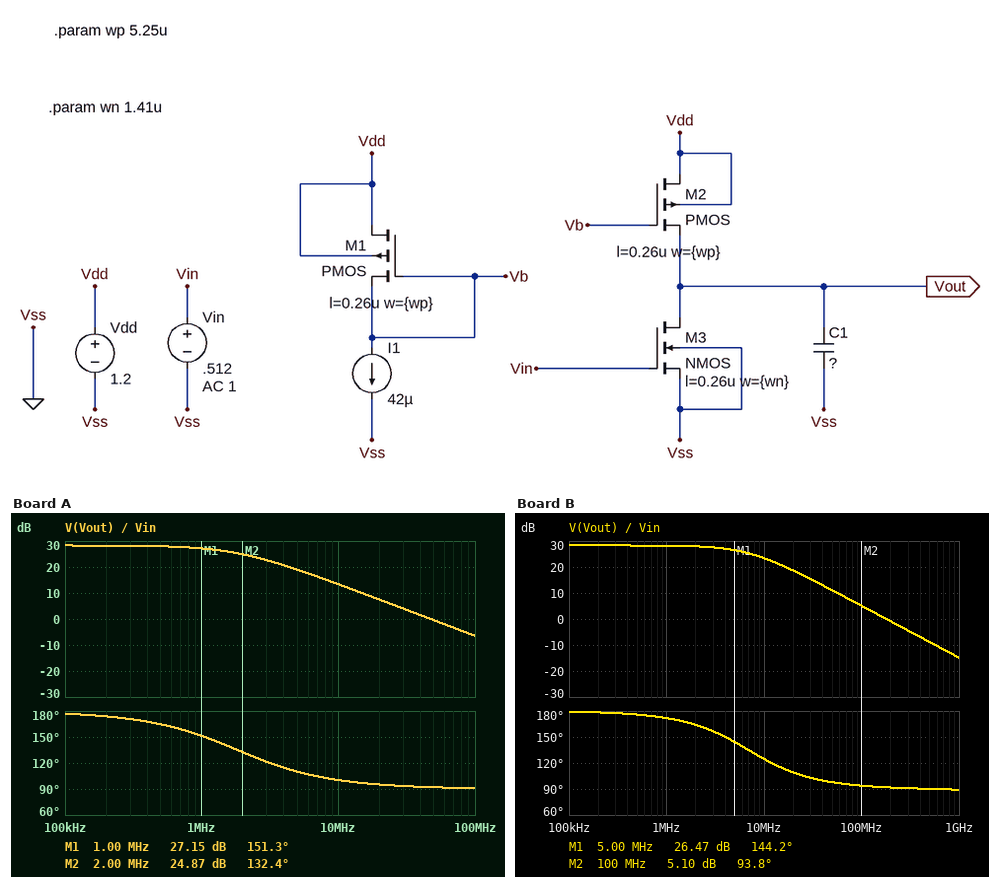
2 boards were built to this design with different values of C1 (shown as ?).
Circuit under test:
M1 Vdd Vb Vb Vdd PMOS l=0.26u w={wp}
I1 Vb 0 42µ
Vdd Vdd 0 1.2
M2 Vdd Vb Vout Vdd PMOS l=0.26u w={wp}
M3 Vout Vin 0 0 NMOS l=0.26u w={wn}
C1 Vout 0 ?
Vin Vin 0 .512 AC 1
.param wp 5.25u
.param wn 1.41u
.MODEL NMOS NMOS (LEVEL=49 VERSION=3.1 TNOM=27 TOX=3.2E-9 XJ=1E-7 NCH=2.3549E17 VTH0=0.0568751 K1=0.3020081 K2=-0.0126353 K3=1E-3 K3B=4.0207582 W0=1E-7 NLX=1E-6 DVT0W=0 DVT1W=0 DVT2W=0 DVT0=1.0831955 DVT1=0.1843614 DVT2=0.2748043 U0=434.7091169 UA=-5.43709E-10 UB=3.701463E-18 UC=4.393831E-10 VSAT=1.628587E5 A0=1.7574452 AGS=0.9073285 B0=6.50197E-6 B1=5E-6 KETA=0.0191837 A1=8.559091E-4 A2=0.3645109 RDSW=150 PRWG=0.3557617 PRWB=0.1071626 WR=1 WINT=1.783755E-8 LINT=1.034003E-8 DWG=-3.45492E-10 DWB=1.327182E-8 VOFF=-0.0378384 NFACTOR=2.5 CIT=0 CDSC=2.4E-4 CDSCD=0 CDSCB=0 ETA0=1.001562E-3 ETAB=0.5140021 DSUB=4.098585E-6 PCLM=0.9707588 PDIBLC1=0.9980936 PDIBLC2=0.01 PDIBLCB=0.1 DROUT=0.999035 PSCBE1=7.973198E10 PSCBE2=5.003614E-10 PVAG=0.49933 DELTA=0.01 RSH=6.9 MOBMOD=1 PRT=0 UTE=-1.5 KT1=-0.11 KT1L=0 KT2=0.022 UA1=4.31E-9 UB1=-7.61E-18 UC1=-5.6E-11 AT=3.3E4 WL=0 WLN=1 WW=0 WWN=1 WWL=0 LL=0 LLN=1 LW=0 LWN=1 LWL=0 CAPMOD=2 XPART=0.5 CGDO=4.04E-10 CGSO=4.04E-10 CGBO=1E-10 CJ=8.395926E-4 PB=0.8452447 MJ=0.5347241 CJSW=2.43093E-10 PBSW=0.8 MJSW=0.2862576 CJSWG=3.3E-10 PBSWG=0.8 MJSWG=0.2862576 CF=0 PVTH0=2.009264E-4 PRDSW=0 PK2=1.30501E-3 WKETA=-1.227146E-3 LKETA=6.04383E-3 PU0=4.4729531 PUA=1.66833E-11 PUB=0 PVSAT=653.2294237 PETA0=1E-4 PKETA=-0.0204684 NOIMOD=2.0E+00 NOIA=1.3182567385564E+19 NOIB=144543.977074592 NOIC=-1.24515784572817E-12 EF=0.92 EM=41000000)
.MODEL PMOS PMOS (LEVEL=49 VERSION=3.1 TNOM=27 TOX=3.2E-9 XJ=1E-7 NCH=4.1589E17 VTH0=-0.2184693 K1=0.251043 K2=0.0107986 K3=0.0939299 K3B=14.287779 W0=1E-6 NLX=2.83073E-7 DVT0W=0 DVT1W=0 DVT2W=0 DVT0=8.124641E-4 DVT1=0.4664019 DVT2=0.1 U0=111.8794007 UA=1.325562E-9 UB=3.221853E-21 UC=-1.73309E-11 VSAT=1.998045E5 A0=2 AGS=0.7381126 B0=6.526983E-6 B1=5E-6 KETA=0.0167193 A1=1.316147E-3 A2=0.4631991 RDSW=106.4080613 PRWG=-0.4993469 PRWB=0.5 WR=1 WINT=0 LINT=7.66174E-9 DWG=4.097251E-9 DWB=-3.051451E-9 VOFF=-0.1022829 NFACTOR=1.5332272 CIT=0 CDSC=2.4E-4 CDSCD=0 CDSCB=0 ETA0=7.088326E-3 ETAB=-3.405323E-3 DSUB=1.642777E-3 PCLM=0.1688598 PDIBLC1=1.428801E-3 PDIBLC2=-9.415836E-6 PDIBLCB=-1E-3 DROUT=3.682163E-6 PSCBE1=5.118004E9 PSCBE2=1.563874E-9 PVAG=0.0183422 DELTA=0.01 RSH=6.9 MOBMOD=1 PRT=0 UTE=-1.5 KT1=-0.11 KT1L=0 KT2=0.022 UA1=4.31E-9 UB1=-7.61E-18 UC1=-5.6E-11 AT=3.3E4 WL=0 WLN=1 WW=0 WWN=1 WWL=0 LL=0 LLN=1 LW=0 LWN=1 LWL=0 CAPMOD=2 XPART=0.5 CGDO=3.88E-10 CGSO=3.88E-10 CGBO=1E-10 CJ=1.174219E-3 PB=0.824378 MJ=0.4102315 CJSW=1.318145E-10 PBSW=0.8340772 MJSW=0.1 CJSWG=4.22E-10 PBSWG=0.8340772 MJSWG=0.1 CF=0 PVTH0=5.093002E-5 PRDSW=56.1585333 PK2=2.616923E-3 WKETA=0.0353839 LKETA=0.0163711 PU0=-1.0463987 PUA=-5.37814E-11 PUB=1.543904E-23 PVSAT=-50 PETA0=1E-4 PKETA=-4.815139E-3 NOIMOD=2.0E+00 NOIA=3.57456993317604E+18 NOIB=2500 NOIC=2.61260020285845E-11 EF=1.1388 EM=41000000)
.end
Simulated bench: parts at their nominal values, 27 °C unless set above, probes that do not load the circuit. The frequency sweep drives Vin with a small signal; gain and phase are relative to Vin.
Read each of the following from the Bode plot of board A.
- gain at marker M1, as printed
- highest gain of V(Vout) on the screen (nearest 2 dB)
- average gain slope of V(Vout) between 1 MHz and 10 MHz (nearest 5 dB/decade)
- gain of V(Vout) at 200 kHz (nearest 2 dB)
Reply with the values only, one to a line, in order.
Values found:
27.15 dB
28 dB
-15 dB/decade
28 dB
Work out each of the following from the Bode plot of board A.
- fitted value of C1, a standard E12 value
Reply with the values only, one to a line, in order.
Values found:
1.5 pF
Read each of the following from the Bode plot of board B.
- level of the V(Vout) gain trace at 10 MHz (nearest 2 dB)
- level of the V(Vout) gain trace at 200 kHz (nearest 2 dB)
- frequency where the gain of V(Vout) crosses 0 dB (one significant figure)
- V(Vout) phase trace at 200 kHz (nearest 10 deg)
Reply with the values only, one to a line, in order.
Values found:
24 dB
28 dB
200 MHz
180 deg
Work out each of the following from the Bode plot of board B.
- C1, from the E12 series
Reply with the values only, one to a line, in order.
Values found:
390 fF
